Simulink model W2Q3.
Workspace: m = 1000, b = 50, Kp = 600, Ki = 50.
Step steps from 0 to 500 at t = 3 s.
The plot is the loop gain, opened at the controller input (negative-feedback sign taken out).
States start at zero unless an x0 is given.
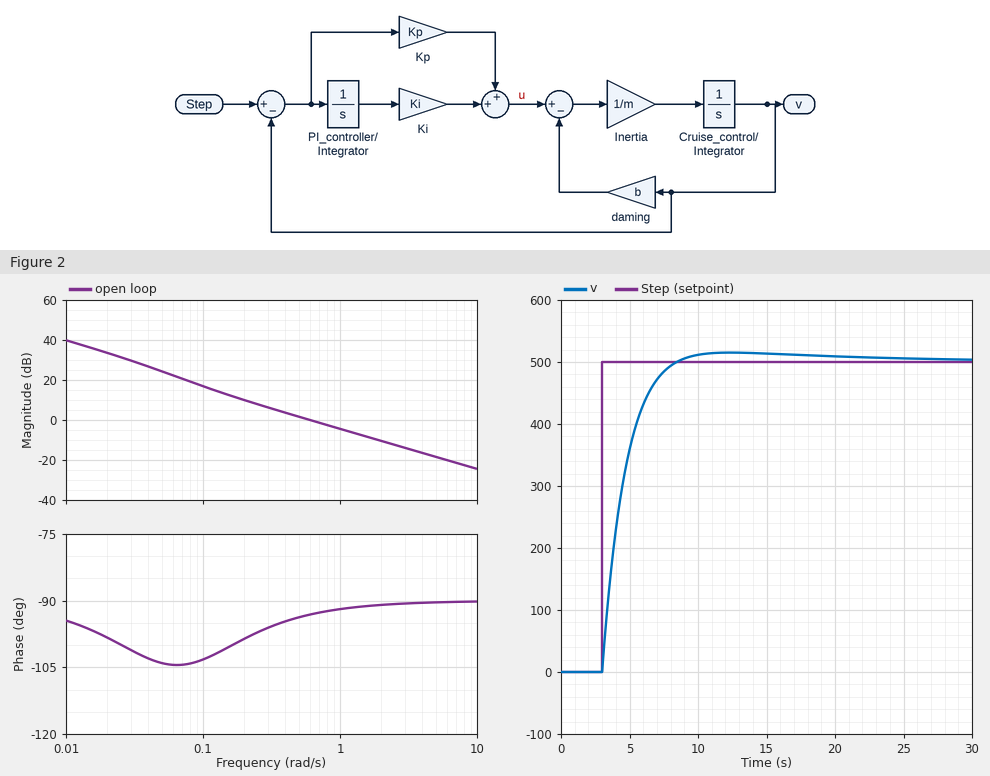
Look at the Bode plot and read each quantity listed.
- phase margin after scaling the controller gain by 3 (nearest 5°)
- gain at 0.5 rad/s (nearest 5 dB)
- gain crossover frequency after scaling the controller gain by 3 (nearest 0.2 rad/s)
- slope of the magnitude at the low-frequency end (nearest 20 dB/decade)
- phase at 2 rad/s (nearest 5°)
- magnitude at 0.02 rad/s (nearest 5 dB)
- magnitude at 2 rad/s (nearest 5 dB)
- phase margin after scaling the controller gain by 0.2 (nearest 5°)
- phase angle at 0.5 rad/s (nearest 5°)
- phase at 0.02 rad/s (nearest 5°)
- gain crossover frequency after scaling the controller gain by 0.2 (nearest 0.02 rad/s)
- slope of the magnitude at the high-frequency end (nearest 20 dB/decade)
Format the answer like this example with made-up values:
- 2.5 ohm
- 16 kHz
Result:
- 90°
- 0 dB
- 1.8 rad/s
- -20 dB/decade
- -90°
- 35 dB
- -10 dB
- 80°
- -95°
- -100°
- 0.14 rad/s
- -20 dB/decade
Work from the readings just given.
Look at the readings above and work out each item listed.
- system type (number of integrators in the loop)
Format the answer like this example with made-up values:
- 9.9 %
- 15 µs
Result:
- 1
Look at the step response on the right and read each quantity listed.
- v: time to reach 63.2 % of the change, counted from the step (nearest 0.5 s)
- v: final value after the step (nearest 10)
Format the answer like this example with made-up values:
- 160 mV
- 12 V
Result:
- 1.5 s
- 500
